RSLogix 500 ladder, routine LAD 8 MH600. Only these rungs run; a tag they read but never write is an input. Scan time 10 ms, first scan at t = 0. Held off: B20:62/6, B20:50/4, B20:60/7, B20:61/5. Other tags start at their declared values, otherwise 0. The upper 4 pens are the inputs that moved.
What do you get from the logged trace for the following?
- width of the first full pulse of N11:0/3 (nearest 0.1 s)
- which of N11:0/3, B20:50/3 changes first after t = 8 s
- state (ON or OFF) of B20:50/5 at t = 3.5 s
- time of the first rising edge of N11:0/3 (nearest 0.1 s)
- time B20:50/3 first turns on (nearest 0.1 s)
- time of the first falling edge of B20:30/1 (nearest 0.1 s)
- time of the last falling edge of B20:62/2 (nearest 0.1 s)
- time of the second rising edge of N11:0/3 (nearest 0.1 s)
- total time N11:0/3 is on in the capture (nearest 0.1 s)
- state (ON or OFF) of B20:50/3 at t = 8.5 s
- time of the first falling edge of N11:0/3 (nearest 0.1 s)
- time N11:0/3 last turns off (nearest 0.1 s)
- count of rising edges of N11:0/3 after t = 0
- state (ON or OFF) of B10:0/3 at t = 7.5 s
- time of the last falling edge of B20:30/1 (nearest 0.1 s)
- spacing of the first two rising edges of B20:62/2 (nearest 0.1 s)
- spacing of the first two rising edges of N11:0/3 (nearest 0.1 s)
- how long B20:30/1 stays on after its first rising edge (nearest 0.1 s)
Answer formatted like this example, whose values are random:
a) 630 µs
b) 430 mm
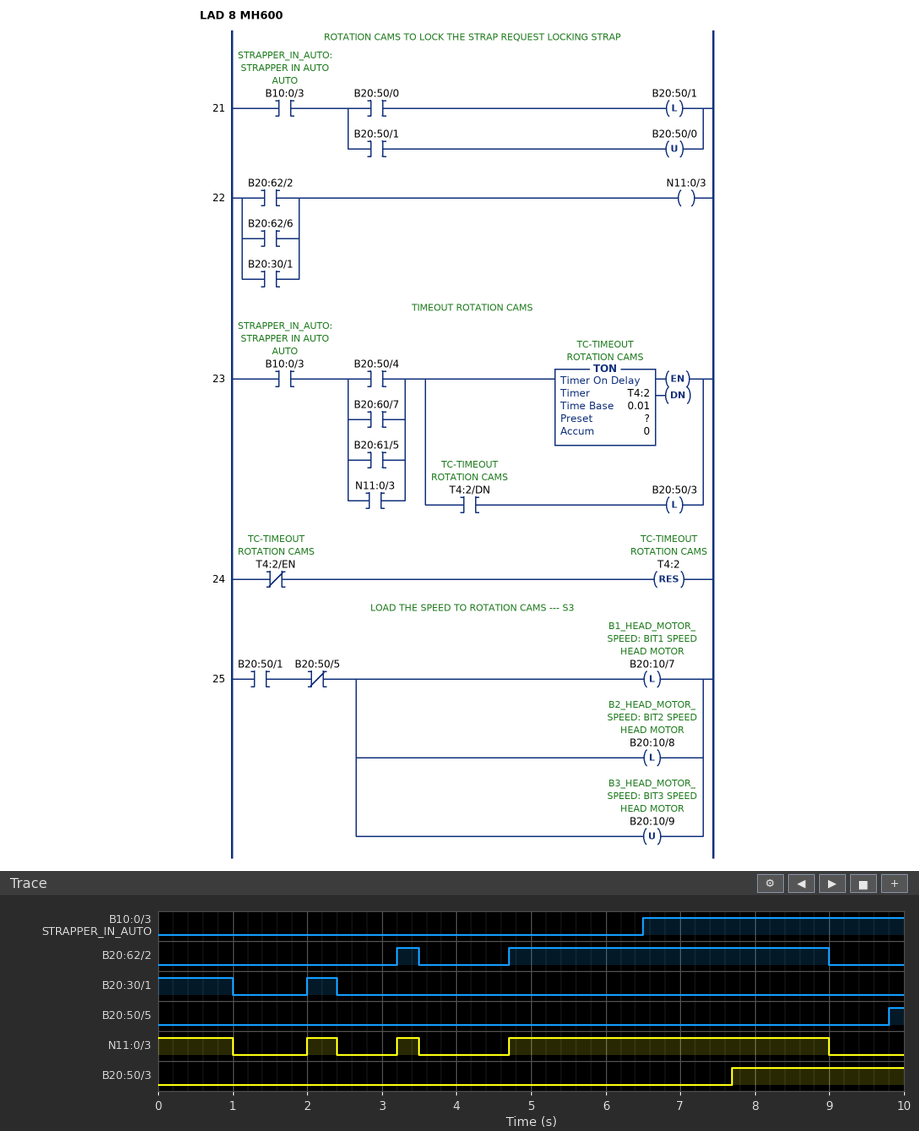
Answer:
a) 0.4 s
b) N11:0/3
c) OFF
d) 2.0 s
e) 7.7 s
f) 1.0 s
g) 9.0 s
h) 3.2 s
i) 6.0 s
j) ON
k) 1.0 s
l) 9.0 s
m) 3
n) ON
o) 2.4 s
p) 1.5 s
q) 1.2 s
r) 0.4 s
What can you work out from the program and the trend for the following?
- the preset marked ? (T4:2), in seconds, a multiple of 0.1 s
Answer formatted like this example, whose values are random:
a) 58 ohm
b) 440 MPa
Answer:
a) 1.2 s
